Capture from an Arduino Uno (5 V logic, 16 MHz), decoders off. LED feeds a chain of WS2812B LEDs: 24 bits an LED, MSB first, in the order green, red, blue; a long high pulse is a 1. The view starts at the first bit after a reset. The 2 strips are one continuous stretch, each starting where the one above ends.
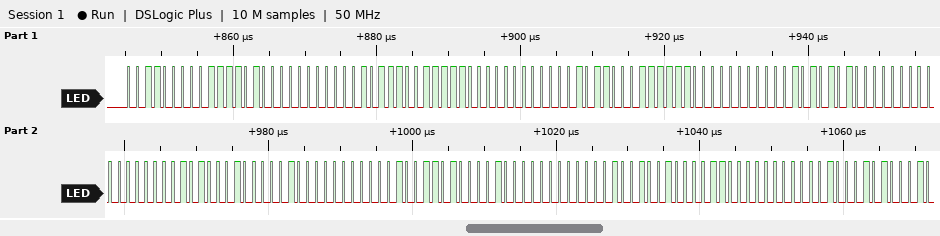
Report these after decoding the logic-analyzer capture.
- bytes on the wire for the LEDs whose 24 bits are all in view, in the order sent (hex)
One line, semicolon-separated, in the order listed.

30 7A 00 2E 7C 00 2C 7E 00 2A 80 00 28 82 00 26 84 00 24 86 00
